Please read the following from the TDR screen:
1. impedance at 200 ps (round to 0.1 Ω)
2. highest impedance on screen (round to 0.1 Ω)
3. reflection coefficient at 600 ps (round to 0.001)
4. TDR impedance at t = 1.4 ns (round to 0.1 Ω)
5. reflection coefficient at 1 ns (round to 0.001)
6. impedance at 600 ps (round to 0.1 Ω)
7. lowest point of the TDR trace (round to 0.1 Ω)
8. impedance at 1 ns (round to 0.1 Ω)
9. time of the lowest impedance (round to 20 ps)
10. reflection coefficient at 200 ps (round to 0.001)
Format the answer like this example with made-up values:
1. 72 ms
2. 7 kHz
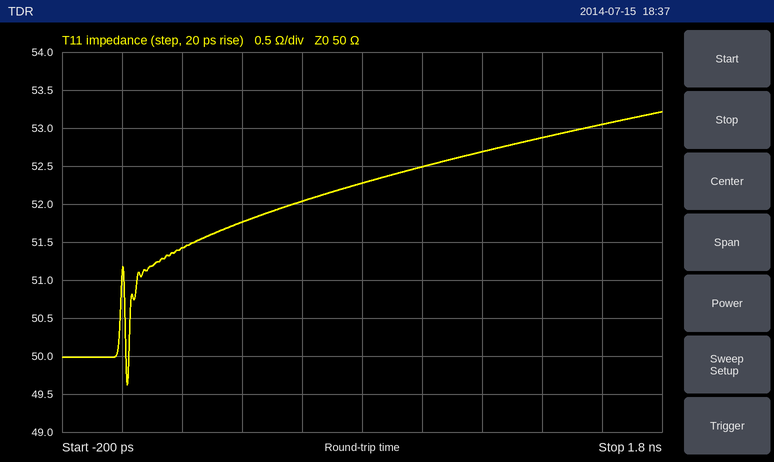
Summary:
1. 51.4 Ω
2. 53.2 Ω
3. +0.020
4. 52.9 Ω
5. +0.024
6. 52.0 Ω
7. 49.6 Ω
8. 52.5 Ω
9. 20 ps
10. +0.014
